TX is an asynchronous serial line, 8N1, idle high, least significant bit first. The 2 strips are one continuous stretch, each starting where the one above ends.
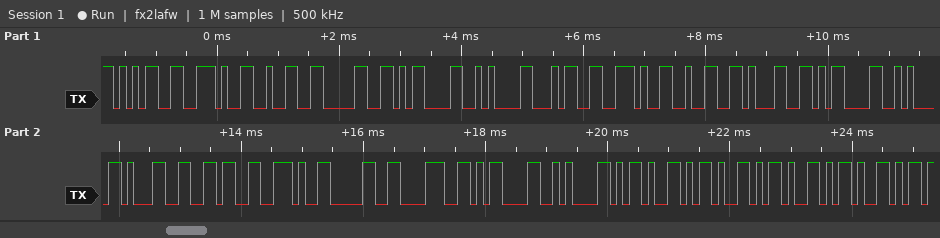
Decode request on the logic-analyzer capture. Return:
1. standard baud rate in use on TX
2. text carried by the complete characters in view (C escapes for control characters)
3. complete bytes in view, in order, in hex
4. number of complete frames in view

9600 baud
"5.20\r\n4.21\r\n16.08\r\n----"
35 2E 32 30 0D 0A 34 2E 32 31 0D 0A 31 36 2E 30 38 0D 0A 2D 2D 2D 2D
23
